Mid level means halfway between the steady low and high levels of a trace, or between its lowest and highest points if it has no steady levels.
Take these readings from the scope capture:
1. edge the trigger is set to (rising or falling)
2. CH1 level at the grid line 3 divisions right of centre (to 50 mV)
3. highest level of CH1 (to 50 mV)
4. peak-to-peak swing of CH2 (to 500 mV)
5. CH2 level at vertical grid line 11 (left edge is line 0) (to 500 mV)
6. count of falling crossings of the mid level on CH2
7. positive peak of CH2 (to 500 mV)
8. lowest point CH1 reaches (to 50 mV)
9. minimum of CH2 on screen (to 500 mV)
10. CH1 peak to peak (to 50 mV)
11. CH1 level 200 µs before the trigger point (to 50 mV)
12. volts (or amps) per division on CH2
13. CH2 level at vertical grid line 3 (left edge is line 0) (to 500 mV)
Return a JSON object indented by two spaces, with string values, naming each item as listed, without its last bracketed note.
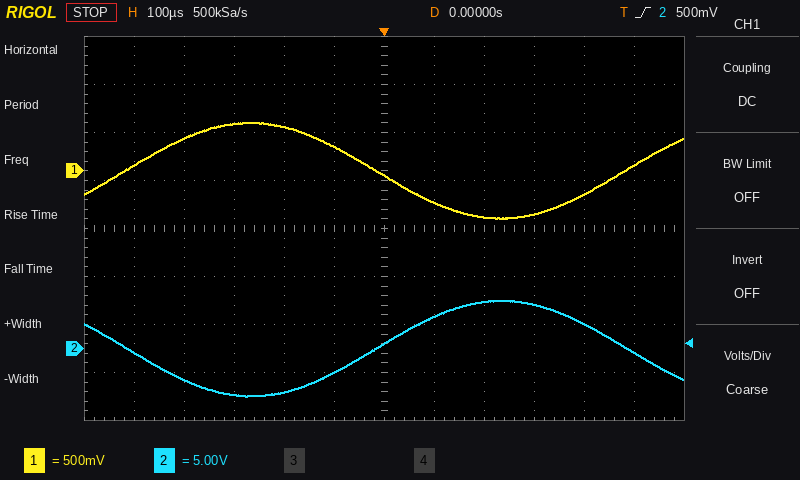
{
  "edge the trigger is set to": "rising",
  "CH1 level at the grid line 3 divisions right of centre": "-450 mV",
  "highest level of CH1": "500 mV",
  "peak-to-peak swing of CH2": "10.0 V",
  "CH2 level at vertical grid line 11 (left edge is line 0)": "-500 mV",
  "count of falling crossings of the mid level on CH2": "2",
  "positive peak of CH2": "5.0 V",
  "lowest point CH1 reaches": "-500 mV",
  "minimum of CH2 on screen": "-5.0 V",
  "CH1 peak to peak": "1.00 V",
  "CH1 level 200 µs before the trigger point": "450 mV",
  "volts (or amps) per division on CH2": "5 V",
  "CH2 level at vertical grid line 3 (left edge is line 0)": "-5.0 V"
}
